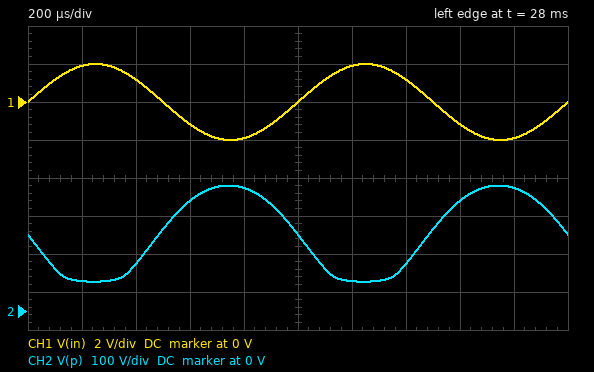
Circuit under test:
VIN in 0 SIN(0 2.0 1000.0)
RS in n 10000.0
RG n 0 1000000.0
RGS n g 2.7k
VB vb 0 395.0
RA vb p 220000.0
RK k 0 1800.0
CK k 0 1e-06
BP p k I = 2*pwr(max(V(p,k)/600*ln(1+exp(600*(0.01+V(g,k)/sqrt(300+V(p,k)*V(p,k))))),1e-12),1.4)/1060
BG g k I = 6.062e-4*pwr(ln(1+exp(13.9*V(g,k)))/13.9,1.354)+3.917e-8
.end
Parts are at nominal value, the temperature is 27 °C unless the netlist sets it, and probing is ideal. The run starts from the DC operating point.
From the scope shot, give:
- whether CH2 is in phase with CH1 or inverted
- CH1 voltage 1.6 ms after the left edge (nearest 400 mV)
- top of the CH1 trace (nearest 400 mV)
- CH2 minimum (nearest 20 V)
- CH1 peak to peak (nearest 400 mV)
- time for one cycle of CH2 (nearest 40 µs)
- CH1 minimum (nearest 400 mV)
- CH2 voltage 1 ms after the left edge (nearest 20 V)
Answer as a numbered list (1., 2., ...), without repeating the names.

1. inverted
2. -1.2 V
3. 2.0 V
4. 80 V
5. 4.0 V
6. 1.00 ms
7. -2.0 V
8. 200 V
